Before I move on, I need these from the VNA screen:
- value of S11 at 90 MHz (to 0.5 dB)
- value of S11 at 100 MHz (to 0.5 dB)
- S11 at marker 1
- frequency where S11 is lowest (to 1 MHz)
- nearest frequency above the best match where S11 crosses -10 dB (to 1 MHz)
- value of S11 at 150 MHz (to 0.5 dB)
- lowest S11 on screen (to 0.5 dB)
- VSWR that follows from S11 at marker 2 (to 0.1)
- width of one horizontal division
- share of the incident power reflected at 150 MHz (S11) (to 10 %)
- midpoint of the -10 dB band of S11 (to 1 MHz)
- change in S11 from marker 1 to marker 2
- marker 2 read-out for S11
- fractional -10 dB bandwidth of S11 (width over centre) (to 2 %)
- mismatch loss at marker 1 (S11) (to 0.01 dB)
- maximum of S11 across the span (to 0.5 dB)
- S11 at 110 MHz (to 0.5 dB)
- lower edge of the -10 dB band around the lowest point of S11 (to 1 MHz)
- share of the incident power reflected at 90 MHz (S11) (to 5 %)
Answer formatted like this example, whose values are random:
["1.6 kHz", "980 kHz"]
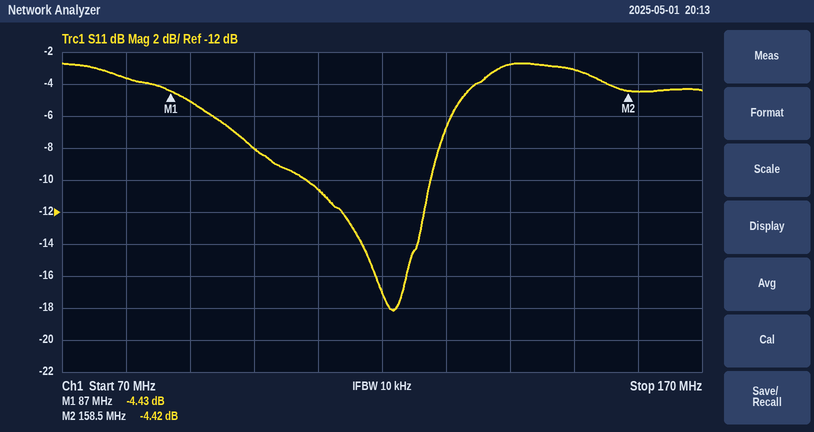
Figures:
["-5.0 dB", "-8.0 dB", "-4.43 dB", "122 MHz", "128 MHz", "-3.0 dB", "-18.0 dB", "4.0", "10 MHz", "50 %", "118 MHz", "0.01 dB", "-4.42 dB", "16 %", "1.94 dB", "-2.5 dB", "-10.5 dB", "108 MHz", "30 %"]
